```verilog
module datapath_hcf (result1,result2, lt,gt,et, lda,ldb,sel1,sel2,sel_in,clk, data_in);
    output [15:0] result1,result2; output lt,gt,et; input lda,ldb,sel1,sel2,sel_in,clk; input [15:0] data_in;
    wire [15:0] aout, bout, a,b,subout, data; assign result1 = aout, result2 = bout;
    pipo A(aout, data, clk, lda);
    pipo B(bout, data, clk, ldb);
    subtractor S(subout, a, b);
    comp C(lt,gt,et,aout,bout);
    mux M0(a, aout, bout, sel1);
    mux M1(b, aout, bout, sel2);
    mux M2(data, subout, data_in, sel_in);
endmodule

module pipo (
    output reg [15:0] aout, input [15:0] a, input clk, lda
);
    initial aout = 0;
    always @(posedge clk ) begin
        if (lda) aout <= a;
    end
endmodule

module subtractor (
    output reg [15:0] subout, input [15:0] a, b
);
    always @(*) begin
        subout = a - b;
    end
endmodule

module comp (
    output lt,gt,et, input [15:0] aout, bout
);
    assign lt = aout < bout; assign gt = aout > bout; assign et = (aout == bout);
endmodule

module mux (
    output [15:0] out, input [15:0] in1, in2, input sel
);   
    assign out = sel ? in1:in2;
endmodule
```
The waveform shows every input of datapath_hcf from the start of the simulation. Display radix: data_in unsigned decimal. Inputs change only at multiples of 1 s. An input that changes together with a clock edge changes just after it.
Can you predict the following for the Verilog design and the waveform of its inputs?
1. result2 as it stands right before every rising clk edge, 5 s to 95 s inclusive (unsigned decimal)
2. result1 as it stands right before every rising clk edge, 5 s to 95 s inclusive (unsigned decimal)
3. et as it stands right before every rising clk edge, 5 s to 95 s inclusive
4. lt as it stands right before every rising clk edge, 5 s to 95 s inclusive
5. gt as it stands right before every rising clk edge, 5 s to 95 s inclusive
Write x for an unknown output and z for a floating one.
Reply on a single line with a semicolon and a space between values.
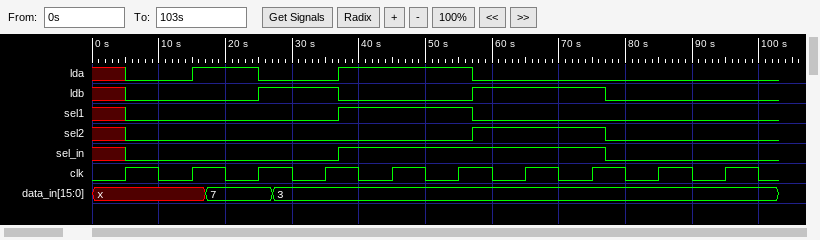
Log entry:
0, 0, 0, 0, 3, 3, 3, 2, 1, 1; 0, 0, 0, 7, 7, 4, 1, 1, 1, 1; 1 1 1 0 0 0 0 0 1 1; 0 0 0 0 0 0 1 1 0 0; 0 0 0 1 1 1 0 0 0 0
